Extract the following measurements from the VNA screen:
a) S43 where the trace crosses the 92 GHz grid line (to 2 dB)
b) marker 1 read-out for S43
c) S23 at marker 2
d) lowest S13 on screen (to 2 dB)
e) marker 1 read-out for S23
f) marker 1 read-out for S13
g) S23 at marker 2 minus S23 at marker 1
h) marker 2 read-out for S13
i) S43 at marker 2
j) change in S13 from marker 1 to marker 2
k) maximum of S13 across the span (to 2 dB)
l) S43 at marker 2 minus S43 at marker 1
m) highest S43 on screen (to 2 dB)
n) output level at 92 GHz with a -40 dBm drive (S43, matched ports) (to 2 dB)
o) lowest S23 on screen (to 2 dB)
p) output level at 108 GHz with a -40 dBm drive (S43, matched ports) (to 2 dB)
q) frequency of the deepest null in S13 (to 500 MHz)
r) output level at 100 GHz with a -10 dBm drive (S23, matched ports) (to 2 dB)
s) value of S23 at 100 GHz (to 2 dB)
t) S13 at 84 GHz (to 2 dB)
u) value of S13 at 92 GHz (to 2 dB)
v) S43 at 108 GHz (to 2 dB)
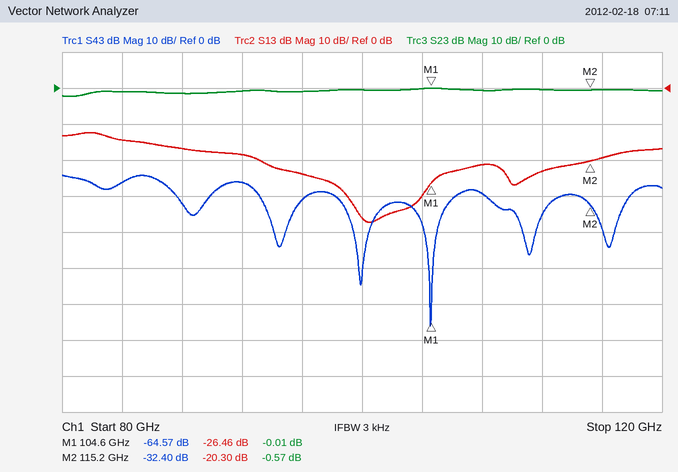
-26 dB
-64.57 dB
-0.57 dB
-38 dB
-0.01 dB
-26.46 dB
-0.56 dB
-20.30 dB
-32.40 dB
6.16 dB
-12 dB
32.17 dB
-24 dB
-66 dBm
-2 dB
-70 dBm
100.5 GHz
-10 dBm
0 dB
-14 dB
-18 dB
-30 dB
